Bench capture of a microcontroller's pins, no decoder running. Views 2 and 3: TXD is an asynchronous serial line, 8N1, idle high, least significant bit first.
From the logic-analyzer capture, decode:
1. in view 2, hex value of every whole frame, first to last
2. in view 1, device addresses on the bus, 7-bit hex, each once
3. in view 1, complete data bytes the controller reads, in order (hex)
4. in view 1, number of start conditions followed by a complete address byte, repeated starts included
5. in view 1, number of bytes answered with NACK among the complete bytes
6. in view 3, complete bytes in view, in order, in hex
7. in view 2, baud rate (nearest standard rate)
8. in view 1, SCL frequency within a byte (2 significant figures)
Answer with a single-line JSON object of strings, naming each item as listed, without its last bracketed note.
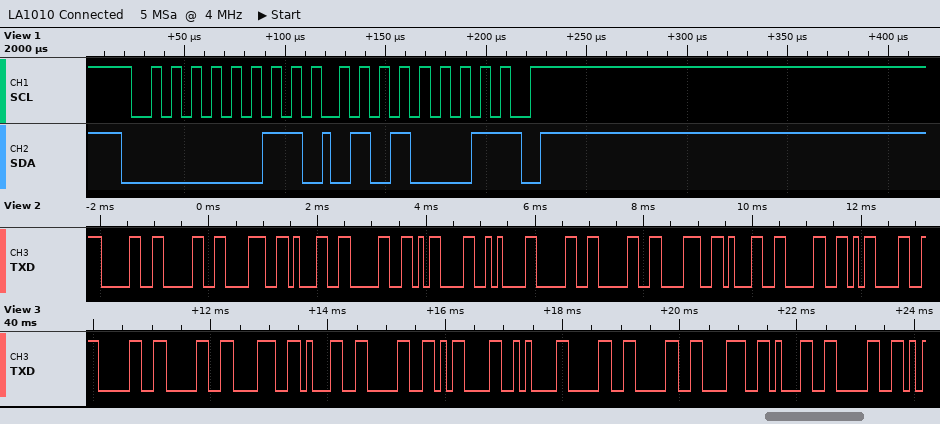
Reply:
{"in view 2, hex value of every whole frame, first to last": "0x30 0x30 0x38 0x31 0x30 0x0D 0x0A 0x30 0x30 0x38 0x31 0x30 0x0D", "in view 1, device addresses on the bus, 7-bit hex, each once": "0x01", "in view 1, complete data bytes the controller reads, in order": "51", "in view 1, number of start conditions followed by a complete address byte, repeated starts included": "1", "in view 1, number of bytes answered with NACK among the complete bytes": "1", "in view 3, complete bytes in view, in order, in hex": "30 30 38 31 30 0D 0A 30 30 38 31 30", "in view 2, baud rate": "9600 baud", "in view 1, SCL frequency within a byte": "100 kHz"}
